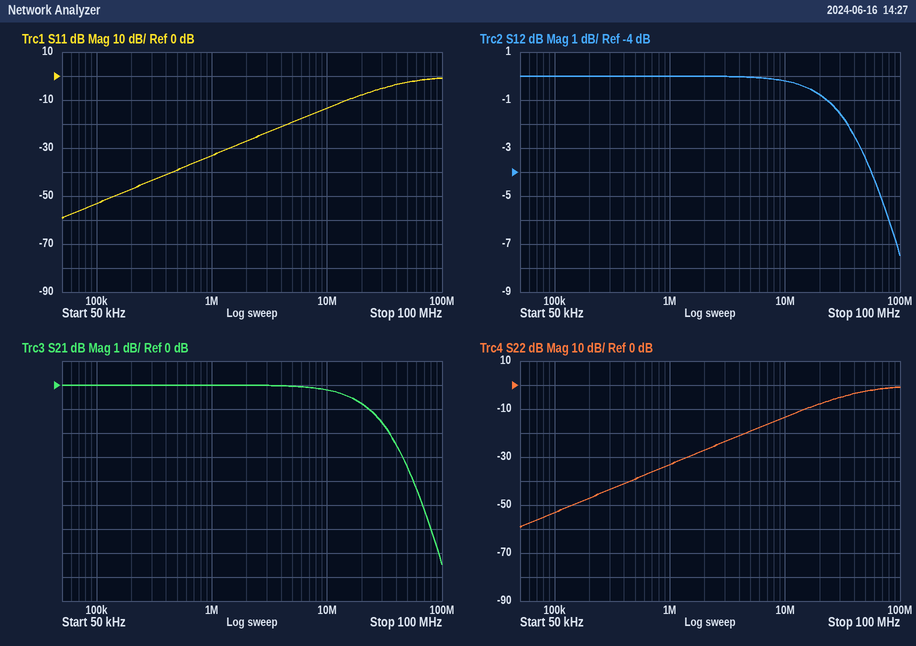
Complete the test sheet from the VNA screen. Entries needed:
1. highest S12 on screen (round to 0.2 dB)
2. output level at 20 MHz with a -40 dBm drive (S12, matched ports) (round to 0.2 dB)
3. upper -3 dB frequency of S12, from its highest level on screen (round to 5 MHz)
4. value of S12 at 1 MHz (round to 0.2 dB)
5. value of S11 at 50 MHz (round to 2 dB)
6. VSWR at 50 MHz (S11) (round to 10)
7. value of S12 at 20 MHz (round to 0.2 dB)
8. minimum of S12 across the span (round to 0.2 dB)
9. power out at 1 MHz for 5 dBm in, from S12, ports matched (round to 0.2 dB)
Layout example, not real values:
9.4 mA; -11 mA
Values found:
0.0 dB; -40.8 dBm; 45 MHz; 0.0 dB; -2 dB; 10; -0.8 dB; -7.4 dB; 5.0 dBm
